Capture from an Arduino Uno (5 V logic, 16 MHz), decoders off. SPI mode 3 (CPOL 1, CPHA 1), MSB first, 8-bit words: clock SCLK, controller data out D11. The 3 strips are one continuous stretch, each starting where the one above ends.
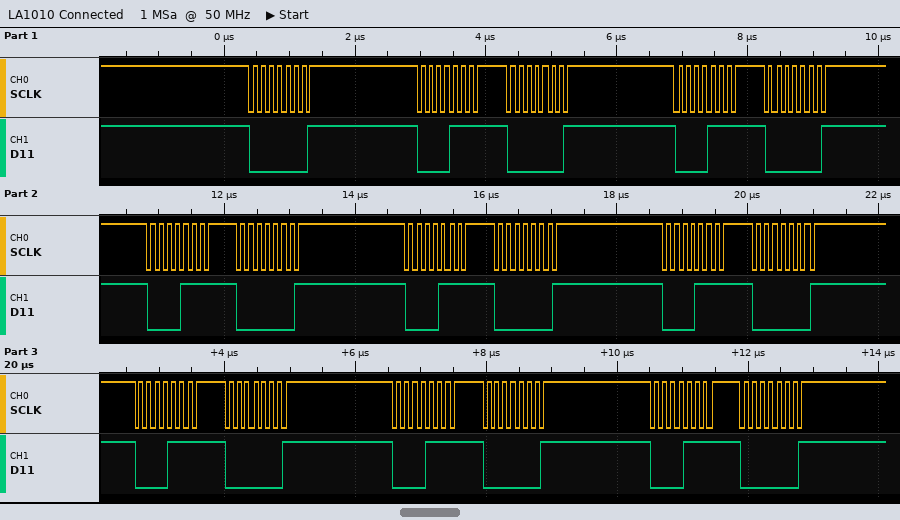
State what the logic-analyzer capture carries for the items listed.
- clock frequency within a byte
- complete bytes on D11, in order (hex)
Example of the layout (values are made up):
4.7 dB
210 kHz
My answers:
8 MHz
01 0F 01 0F 01 0F 01 0F 01 0F 01 0F 01 0F 01 0F 01
